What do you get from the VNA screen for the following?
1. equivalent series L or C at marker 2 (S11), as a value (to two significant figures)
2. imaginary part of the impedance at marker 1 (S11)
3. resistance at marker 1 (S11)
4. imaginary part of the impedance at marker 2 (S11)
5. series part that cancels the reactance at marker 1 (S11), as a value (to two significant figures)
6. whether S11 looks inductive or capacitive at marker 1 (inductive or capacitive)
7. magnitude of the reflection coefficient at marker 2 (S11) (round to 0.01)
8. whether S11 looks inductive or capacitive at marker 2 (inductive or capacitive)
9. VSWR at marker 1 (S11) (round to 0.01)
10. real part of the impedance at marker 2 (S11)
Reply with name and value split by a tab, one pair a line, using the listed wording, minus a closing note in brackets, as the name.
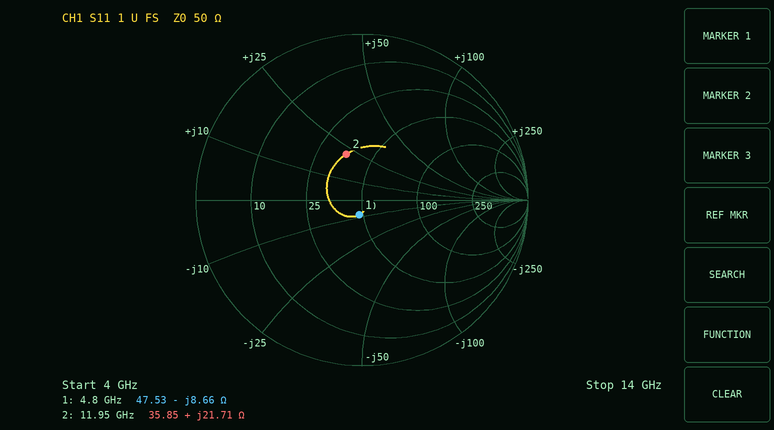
equivalent series L or C at marker 2 (S11), as a value	290 pH
imaginary part of the impedance at marker 1	-8.66 Ω
resistance at marker 1	47.53 Ω
imaginary part of the impedance at marker 2	+21.71 Ω
series part that cancels the reactance at marker 1 (S11), as a value	290 pH
whether S11 looks inductive or capacitive at marker 1	capacitive
magnitude of the reflection coefficient at marker 2 (S11)	0.29
whether S11 looks inductive or capacitive at marker 2	inductive
VSWR at marker 1 (S11)	1.20
real part of the impedance at marker 2	35.85 Ω
